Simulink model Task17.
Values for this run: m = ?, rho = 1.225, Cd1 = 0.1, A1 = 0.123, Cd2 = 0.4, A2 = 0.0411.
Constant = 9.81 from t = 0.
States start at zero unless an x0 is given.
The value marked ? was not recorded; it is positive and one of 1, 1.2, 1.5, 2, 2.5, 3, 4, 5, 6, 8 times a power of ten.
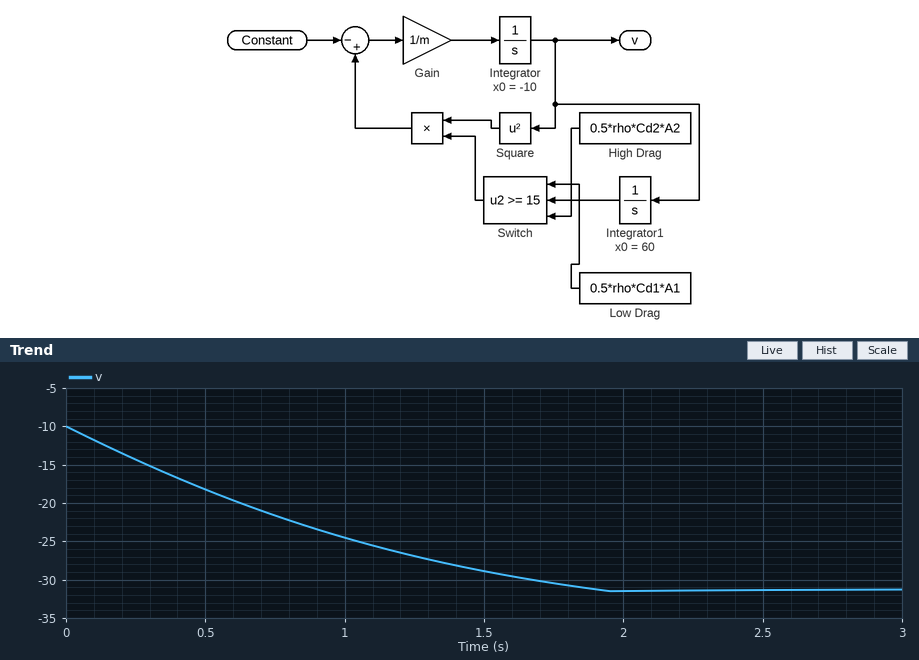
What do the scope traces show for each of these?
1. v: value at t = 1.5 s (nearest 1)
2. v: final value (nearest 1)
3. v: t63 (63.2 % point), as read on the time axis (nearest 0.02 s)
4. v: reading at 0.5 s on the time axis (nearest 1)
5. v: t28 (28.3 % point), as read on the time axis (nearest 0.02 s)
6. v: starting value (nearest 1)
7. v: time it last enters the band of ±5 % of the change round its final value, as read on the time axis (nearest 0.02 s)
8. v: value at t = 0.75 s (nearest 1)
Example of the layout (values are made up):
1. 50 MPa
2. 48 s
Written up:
1. -29
2. -31
3. 0.90 s
4. -18
5. 0.36 s
6. -10
7. 1.70 s
8. -22
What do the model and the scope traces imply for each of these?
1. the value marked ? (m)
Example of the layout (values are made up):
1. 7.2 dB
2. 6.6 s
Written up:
1. 0.5
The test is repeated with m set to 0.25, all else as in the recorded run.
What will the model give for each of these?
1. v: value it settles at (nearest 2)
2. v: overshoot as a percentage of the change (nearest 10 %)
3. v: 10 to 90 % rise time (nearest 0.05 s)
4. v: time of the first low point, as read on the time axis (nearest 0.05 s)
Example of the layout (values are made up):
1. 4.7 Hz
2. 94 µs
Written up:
1. -32
2. 20 %
3. 0.70 s
4. 1.65 s
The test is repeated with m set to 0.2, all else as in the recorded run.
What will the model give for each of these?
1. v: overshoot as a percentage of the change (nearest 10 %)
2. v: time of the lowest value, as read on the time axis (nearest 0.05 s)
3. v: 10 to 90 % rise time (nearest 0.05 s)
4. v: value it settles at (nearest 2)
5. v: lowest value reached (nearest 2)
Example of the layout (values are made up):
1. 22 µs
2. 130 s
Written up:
1. 20 %
2. 1.55 s
3. 0.55 s
4. -32
5. -36
